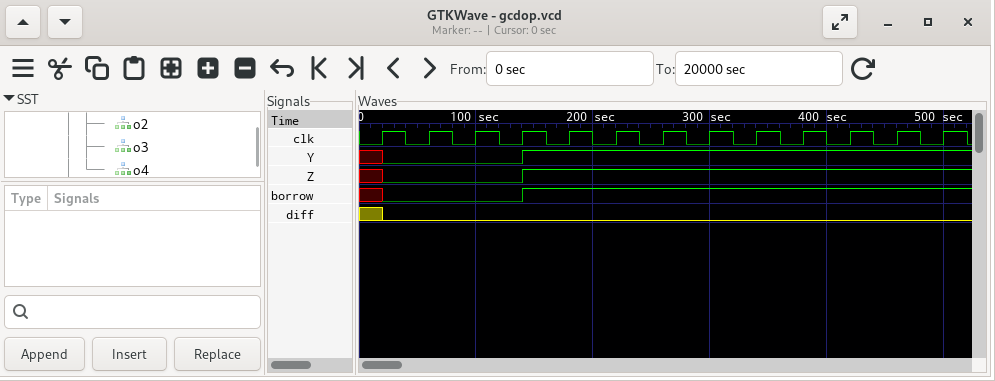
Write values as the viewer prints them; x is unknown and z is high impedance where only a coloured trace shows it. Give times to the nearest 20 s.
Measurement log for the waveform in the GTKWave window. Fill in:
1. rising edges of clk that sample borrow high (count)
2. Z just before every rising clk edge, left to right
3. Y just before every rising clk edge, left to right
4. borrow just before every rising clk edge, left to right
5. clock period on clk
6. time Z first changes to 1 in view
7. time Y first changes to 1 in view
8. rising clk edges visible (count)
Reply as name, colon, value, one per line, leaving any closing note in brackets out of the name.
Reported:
rising edges of clk that sample borrow high: 9
Z just before every rising clk edge, left to right: x 0 0 0 1 1 1 1 1 1 1 1 1
Y just before every rising clk edge, left to right: x 0 0 0 1 1 1 1 1 1 1 1 1
borrow just before every rising clk edge, left to right: x 0 0 0 1 1 1 1 1 1 1 1 1
clock period on clk: 40 s
time Z first changes to 1 in view: 140 s
time Y first changes to 1 in view: 140 s
rising clk edges visible: 13
